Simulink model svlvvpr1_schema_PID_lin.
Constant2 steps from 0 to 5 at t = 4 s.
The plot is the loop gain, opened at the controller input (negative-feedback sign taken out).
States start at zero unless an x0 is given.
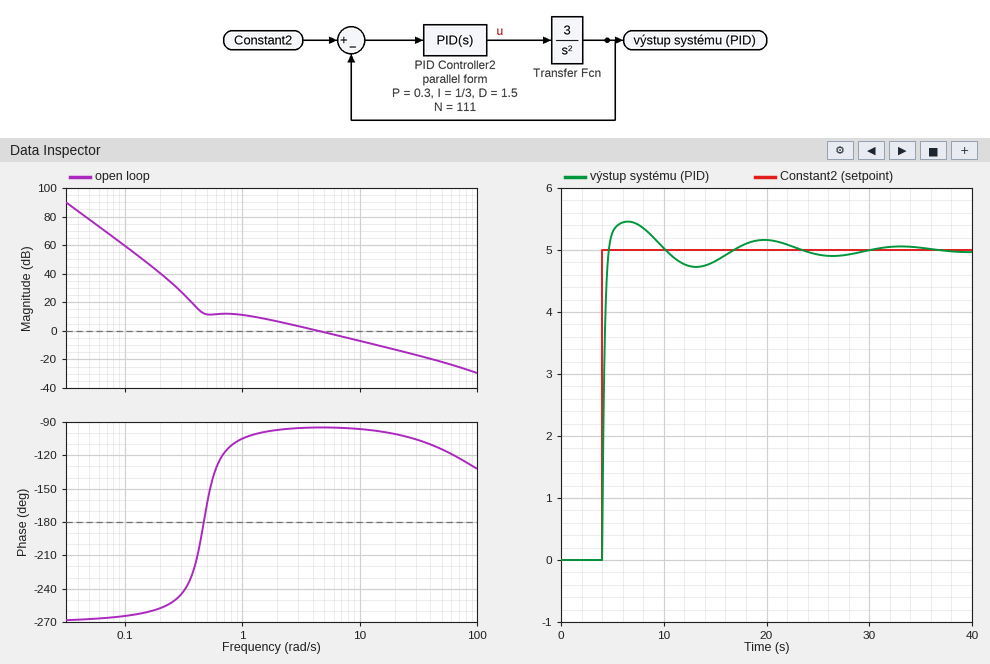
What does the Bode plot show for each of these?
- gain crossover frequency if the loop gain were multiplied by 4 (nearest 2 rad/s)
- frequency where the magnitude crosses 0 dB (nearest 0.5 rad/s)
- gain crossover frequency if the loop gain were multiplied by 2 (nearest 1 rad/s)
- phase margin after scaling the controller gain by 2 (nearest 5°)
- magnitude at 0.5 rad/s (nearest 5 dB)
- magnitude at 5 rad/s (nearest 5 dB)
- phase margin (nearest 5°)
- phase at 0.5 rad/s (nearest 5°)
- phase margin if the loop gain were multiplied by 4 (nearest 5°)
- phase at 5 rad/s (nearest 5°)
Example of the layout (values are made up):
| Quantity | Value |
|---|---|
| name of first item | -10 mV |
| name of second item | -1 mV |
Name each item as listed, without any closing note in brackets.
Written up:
| Quantity | Value |
|---|---|
| gain crossover frequency if the loop gain were multiplied by 4 | 18 rad/s |
| frequency where the magnitude crosses 0 dB | 4.5 rad/s |
| gain crossover frequency if the loop gain were multiplied by 2 | 9 rad/s |
| phase margin after scaling the controller gain by 2 | 85° |
| magnitude at 0.5 rad/s | 10 dB |
| magnitude at 5 rad/s | 0 dB |
| phase margin | 85° |
| phase at 0.5 rad/s | -165° |
| phase margin if the loop gain were multiplied by 4 | 80° |
| phase at 5 rad/s | -95° |
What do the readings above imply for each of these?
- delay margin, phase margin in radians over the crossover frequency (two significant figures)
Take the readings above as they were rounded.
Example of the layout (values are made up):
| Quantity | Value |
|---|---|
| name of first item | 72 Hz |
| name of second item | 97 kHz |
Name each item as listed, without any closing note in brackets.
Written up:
| Quantity | Value |
|---|---|
| delay margin, phase margin in radians over the crossover frequency | 0.33 s |
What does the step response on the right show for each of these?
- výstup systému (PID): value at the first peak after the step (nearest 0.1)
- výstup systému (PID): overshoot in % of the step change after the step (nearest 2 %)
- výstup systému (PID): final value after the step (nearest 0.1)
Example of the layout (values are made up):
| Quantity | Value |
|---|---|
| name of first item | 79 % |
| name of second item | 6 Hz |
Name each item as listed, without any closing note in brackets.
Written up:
| Quantity | Value |
|---|---|
| výstup systému (PID): value at the first peak after the step | 5.5 |
| výstup systému (PID): overshoot in % of the step change after the step | 10 % |
| výstup systému (PID): final value after the step | 5.0 |
